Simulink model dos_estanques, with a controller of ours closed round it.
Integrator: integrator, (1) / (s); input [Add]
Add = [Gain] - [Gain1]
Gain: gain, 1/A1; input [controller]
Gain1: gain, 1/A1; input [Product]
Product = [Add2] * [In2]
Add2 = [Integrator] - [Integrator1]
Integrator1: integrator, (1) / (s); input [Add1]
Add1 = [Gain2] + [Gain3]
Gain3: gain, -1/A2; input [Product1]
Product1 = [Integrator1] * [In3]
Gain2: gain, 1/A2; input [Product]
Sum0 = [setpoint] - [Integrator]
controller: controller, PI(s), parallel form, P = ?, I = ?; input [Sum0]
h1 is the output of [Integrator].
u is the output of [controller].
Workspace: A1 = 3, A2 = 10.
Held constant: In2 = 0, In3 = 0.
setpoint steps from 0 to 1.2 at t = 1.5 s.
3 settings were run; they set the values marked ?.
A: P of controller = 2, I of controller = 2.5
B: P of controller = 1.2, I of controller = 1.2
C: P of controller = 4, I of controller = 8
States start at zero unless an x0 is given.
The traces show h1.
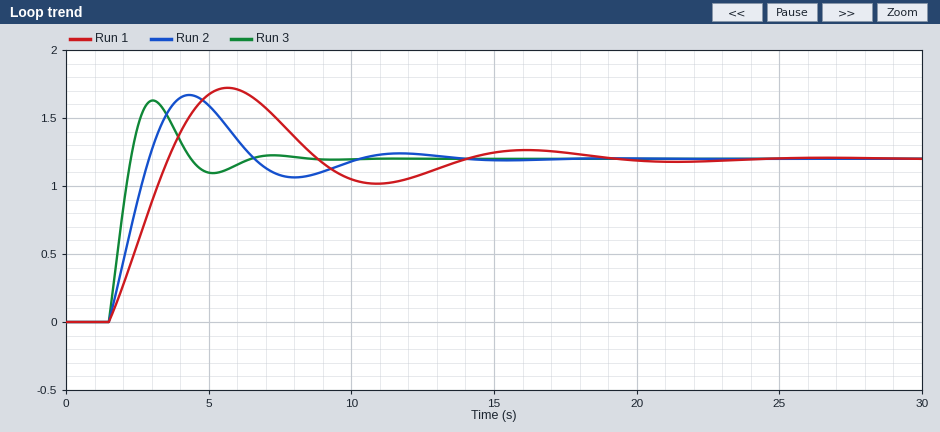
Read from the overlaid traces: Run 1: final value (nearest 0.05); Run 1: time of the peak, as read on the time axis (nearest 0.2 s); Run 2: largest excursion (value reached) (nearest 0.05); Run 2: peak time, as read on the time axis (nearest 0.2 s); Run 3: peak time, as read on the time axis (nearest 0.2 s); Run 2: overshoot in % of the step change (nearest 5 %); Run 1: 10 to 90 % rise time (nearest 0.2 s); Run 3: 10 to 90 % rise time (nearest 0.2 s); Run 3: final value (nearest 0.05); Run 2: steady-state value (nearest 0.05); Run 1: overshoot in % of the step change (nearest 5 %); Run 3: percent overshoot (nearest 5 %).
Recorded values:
1.20
5.6 s
1.65
4.4 s
3.0 s
40 %
1.6 s
0.6 s
1.20
1.20
45 %
35 %
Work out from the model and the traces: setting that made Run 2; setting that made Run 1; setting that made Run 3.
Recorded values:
A
B
C
